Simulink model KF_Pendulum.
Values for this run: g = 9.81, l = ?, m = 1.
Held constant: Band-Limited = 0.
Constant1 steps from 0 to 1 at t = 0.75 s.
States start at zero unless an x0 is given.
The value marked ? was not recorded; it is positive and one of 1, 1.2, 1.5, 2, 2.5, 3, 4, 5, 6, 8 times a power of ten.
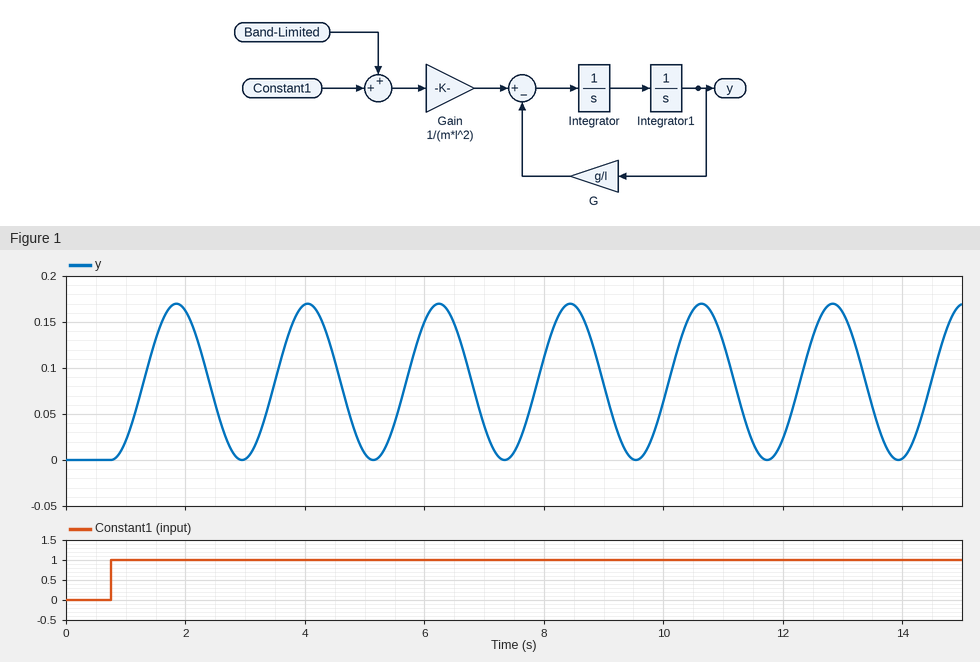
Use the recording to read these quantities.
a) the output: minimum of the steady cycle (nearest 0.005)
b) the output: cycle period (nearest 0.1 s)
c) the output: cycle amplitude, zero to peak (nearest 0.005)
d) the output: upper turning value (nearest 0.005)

0.000
2.2 s
0.085
0.170
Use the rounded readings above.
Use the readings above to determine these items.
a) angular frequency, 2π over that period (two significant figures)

2.9 rad/s
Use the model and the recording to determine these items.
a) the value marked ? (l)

1.2
